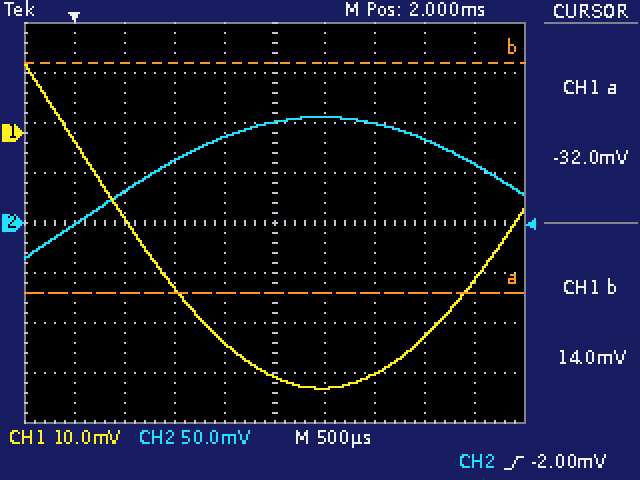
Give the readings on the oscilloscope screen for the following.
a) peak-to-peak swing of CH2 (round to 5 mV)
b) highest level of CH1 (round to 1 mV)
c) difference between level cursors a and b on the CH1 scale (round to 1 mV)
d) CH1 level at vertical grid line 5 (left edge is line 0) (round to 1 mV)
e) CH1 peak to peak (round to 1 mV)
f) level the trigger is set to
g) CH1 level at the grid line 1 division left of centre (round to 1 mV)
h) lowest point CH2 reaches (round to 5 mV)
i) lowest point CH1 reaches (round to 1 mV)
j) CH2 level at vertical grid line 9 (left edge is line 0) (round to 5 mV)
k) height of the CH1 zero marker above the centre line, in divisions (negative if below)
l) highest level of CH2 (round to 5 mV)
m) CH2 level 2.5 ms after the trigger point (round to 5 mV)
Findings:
140 mV
14 mV
46 mV
-49 mV
65 mV
-2.00 mV
-42 mV
-35 mV
-51 mV
60 mV
+1.8 div
105 mV
105 mV
